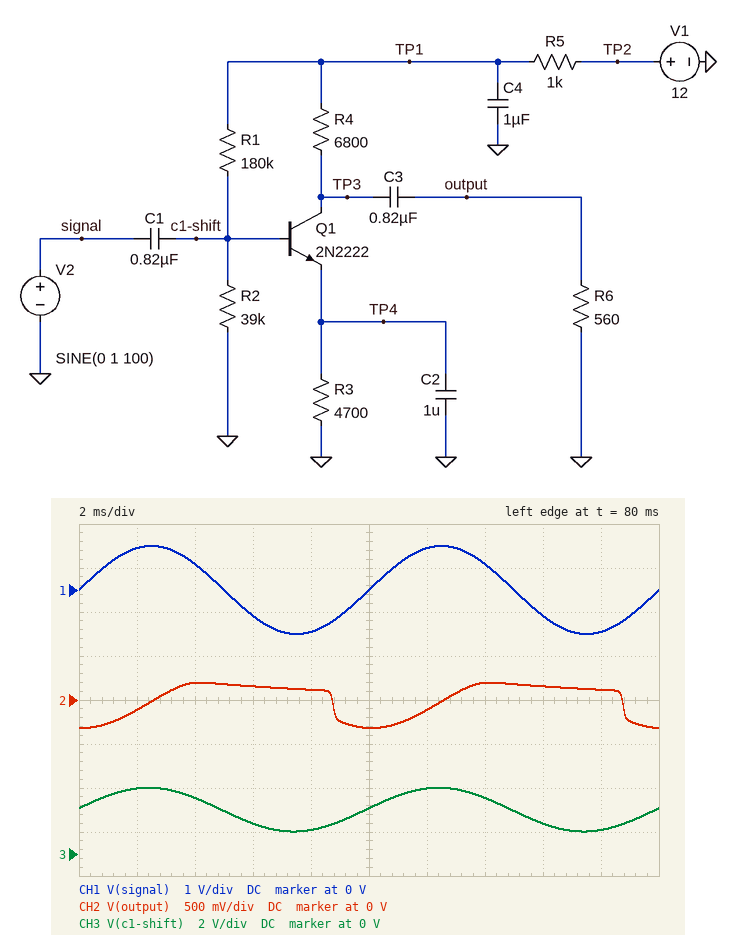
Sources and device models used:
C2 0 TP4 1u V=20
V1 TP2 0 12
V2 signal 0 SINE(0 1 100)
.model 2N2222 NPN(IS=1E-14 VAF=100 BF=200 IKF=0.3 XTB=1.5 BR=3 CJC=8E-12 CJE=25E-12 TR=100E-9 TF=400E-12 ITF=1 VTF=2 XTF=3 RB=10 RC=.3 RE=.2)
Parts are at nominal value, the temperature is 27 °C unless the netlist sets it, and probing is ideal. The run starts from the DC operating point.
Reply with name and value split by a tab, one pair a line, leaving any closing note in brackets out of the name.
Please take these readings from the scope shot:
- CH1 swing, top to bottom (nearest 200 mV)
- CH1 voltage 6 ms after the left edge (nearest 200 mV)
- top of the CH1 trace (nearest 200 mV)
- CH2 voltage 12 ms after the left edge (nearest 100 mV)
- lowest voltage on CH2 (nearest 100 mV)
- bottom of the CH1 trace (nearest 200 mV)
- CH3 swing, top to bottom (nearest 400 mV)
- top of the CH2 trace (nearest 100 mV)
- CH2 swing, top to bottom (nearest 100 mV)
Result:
CH1 swing, top to bottom	2.0 V
CH1 voltage 6 ms after the left edge	-600 mV
top of the CH1 trace	1.0 V
CH2 voltage 12 ms after the left edge	-100 mV
lowest voltage on CH2	-300 mV
bottom of the CH1 trace	-1.0 V
CH3 swing, top to bottom	2.0 V
top of the CH2 trace	200 mV
CH2 swing, top to bottom	500 mV
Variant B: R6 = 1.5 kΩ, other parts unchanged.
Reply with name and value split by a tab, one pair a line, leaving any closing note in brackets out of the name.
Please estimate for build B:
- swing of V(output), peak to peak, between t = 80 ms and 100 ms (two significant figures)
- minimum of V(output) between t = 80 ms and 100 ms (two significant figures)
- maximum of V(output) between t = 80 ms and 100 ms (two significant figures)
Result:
swing of V(output), peak to peak, between t = 80 ms and 100 ms	1.2 V
minimum of V(output) between t = 80 ms and 100 ms	-770 mV
maximum of V(output) between t = 80 ms and 100 ms	470 mV
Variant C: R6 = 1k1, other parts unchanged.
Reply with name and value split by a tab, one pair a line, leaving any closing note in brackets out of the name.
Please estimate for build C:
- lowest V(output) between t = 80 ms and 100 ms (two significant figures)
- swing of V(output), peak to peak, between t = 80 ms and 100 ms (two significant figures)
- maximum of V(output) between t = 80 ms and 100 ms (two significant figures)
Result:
lowest V(output) between t = 80 ms and 100 ms	-590 mV
swing of V(output), peak to peak, between t = 80 ms and 100 ms	950 mV
maximum of V(output) between t = 80 ms and 100 ms	360 mV
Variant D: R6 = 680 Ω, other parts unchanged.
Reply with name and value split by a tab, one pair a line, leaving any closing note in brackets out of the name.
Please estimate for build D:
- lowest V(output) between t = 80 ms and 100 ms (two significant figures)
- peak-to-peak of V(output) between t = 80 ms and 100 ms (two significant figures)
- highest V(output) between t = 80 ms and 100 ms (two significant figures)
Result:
lowest V(output) between t = 80 ms and 100 ms	-380 mV
peak-to-peak of V(output) between t = 80 ms and 100 ms	620 mV
highest V(output) between t = 80 ms and 100 ms	240 mV
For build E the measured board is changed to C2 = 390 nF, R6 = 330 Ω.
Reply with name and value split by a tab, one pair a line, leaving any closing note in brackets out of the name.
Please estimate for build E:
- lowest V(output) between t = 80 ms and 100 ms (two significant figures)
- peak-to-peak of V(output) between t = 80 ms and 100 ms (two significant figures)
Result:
lowest V(output) between t = 80 ms and 100 ms	-96 mV
peak-to-peak of V(output) between t = 80 ms and 100 ms	180 mV
